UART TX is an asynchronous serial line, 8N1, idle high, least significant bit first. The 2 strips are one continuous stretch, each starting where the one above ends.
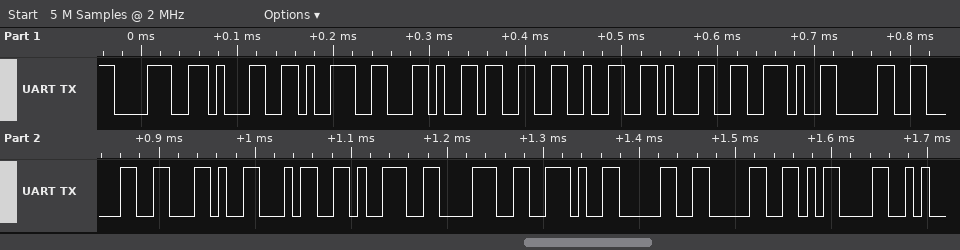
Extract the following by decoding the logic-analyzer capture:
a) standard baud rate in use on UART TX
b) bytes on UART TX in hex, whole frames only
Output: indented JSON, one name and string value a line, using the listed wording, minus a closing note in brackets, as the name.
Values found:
{
  "standard baud rate in use on UART TX": "115200 baud",
  "bytes on UART TX in hex, whole frames only": "38 31 39 2C 33 32 31 2E 30 30 2C 34 39 38 2E 30 30 0D"
}
